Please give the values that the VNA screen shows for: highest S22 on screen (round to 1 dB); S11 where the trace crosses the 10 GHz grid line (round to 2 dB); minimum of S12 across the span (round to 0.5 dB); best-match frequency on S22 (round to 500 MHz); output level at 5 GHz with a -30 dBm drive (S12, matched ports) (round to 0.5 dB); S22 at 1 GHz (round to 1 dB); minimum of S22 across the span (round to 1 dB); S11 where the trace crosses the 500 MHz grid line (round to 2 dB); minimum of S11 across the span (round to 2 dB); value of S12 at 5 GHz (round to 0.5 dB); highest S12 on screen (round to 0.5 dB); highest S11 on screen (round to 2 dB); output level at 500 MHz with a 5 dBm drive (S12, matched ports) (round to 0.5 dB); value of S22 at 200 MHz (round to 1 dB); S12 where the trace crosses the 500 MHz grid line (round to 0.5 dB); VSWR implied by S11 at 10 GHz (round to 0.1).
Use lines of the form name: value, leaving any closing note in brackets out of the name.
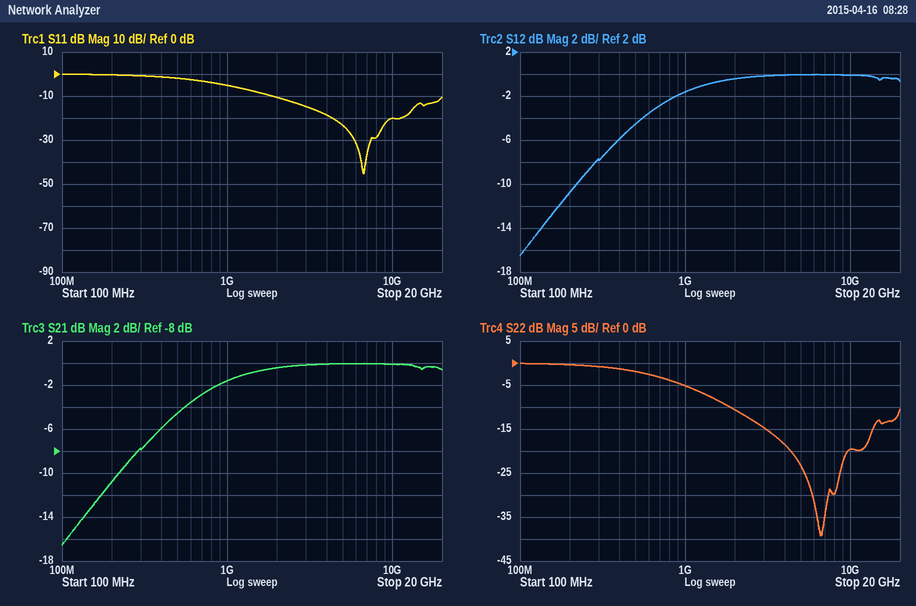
highest S22 on screen: 0 dB
S11 where the trace crosses the 10 GHz grid line: -20 dB
minimum of S12 across the span: -16.5 dB
best-match frequency on S22: 6.5 GHz
output level at 5 GHz with a -30 dBm drive (S12, matched ports): -30.0 dBm
S22 at 1 GHz: -5 dB
minimum of S22 across the span: -39 dB
S11 where the trace crosses the 500 MHz grid line: -2 dB
minimum of S11 across the span: -46 dB
value of S12 at 5 GHz: 0.0 dB
highest S12 on screen: 0.0 dB
highest S11 on screen: 0 dB
output level at 500 MHz with a 5 dBm drive (S12, matched ports): 0.5 dBm
value of S22 at 200 MHz: 0 dB
S12 where the trace crosses the 500 MHz grid line: -4.5 dB
VSWR implied by S11 at 10 GHz: 1.2
